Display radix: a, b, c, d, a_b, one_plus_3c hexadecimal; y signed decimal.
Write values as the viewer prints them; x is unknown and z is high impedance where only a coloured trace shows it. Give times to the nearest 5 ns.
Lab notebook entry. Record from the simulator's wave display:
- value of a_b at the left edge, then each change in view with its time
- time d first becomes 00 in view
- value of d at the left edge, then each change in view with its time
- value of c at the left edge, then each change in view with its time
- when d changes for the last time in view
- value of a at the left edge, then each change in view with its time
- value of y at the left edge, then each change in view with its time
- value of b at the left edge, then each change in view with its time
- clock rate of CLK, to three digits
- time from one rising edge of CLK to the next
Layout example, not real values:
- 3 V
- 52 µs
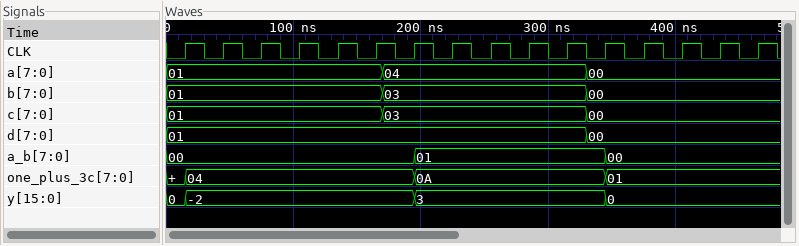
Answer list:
- 00, 01 at 195 ns, 00 at 345 ns
- 330 ns
- 01, 00 at 330 ns
- 01, 03 at 170 ns, 00 at 330 ns
- 330 ns
- 01, 04 at 170 ns, 00 at 330 ns
- 0, -2 at 15 ns, 3 at 195 ns, 0 at 345 ns
- 01, 03 at 170 ns, 00 at 330 ns
- 33.3 MHz
- 30 ns
